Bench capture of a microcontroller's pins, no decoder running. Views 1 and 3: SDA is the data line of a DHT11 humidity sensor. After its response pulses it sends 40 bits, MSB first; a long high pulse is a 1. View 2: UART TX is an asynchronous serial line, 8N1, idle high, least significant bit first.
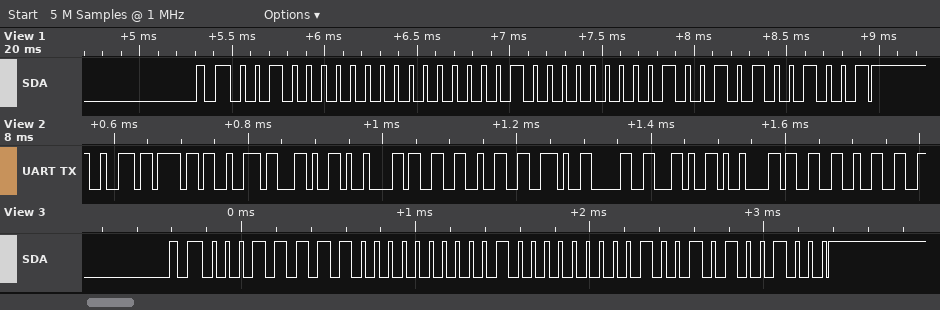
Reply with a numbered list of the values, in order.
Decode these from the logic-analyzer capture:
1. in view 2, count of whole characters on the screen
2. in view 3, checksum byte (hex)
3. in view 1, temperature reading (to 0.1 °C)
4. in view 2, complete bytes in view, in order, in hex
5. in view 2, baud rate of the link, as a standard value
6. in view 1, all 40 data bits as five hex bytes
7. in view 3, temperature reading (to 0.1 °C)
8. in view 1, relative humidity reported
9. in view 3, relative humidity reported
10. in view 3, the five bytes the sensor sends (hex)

1. 13
2. 0x48
3. 32.9 °C
4. 72 6F 72 2C 09 33 32 2E 30 2C 09 33 32
5. 115200 baud
6. 20 00 20 09 49
7. 32.9 °C
8. 32 %
9. 31 %
10. 1F 00 20 09 48
